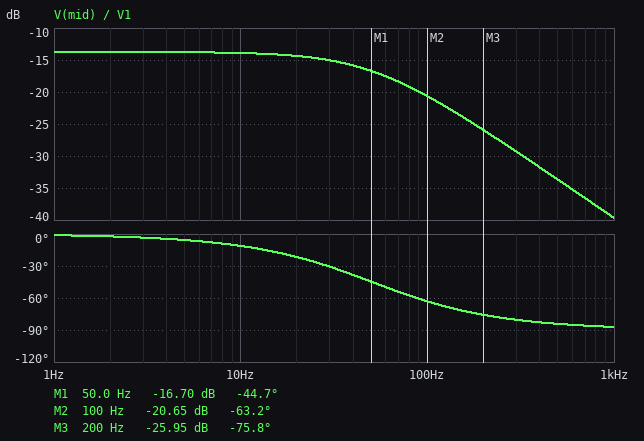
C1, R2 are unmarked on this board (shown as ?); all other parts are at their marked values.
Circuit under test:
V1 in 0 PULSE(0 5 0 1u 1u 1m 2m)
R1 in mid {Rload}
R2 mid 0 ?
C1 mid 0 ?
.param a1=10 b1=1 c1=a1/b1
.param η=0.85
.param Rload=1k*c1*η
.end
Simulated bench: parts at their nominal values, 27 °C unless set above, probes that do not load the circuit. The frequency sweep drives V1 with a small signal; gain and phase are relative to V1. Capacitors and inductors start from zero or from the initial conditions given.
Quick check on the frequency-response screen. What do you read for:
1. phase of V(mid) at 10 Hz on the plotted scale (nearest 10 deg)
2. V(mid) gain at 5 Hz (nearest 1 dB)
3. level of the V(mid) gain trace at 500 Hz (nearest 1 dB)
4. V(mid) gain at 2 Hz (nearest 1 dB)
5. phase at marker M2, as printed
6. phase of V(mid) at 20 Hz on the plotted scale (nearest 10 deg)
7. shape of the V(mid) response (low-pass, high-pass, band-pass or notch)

-10 deg
-14 dB
-34 dB
-14 dB
-63.2 deg
-20 deg
low-pass
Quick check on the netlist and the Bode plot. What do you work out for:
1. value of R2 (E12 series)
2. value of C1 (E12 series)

2.2 kΩ
1.8 µF
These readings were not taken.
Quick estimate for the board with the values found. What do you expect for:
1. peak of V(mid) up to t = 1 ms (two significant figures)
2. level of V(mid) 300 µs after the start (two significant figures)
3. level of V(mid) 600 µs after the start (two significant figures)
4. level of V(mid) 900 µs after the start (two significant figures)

280 mV
93 mV
180 mV
260 mV
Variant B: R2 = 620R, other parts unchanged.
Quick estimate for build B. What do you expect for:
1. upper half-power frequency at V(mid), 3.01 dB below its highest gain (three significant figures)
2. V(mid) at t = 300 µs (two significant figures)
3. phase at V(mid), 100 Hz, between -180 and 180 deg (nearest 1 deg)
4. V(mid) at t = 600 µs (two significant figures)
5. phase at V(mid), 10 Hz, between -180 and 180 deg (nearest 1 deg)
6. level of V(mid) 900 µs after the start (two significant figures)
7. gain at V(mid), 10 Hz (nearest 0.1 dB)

153 Hz
85 mV
-33 deg
150 mV
-4 deg
200 mV
-23.4 dB
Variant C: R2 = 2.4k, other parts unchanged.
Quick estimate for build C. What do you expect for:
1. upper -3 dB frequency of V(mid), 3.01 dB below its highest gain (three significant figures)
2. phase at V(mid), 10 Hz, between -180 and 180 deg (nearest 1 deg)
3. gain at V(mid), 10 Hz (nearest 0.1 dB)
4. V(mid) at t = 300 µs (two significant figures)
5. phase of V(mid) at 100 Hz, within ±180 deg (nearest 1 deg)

47.2 Hz
-12 deg
-13.3 dB
94 mV
-65 deg
